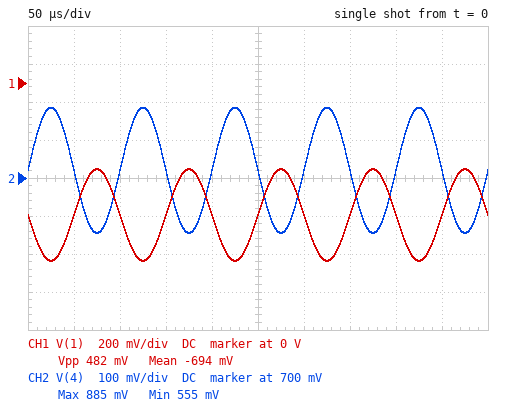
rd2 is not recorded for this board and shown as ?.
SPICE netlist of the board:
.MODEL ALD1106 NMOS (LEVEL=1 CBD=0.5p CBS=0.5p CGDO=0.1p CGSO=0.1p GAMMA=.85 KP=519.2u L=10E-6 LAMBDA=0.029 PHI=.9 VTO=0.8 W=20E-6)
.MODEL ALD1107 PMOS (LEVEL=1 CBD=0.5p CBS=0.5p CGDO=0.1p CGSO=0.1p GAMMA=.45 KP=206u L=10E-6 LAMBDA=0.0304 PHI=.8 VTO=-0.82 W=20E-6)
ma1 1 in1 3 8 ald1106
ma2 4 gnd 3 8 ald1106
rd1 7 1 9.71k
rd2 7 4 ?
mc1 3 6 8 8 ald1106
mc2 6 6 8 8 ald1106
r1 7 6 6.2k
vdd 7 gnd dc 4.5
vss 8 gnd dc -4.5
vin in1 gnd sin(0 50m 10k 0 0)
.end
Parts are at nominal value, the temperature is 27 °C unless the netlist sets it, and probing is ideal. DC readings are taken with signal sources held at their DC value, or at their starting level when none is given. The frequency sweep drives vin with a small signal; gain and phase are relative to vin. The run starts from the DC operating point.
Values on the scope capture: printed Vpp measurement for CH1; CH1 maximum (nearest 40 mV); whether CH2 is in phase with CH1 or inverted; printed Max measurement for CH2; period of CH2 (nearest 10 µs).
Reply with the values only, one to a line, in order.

482 mV
-440 mV
inverted
885 mV
100 µs
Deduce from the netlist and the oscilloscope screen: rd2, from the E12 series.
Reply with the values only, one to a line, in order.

6.8 kΩ
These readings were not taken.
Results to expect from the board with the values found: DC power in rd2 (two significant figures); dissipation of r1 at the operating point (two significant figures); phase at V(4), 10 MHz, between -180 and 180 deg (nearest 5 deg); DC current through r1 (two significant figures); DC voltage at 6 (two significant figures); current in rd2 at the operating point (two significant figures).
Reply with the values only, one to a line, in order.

2.1 mW
7.4 mW
-5 deg
1.1 mA
-2.3 V
560 µA
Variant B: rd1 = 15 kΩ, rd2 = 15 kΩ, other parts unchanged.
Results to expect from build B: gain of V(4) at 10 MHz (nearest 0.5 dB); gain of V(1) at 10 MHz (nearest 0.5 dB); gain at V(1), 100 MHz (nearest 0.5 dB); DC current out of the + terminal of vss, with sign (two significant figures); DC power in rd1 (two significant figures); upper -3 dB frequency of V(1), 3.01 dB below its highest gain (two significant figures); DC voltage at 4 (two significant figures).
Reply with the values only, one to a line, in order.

-34.5 dB
-20.0 dB
-20.5 dB
-2.1 mA
3.9 mW
1.1 GHz
-3.1 V
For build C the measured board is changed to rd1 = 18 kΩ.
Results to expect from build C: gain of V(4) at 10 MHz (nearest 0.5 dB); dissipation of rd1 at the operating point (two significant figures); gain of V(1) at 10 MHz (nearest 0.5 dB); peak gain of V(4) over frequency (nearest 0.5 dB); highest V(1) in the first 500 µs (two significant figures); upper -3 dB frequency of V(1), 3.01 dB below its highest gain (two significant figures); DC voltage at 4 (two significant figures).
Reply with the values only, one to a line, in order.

-16.0 dB
2.5 mW
-7.5 dB
-10.0 dB
-2.2 V
330 MHz
-370 mV
